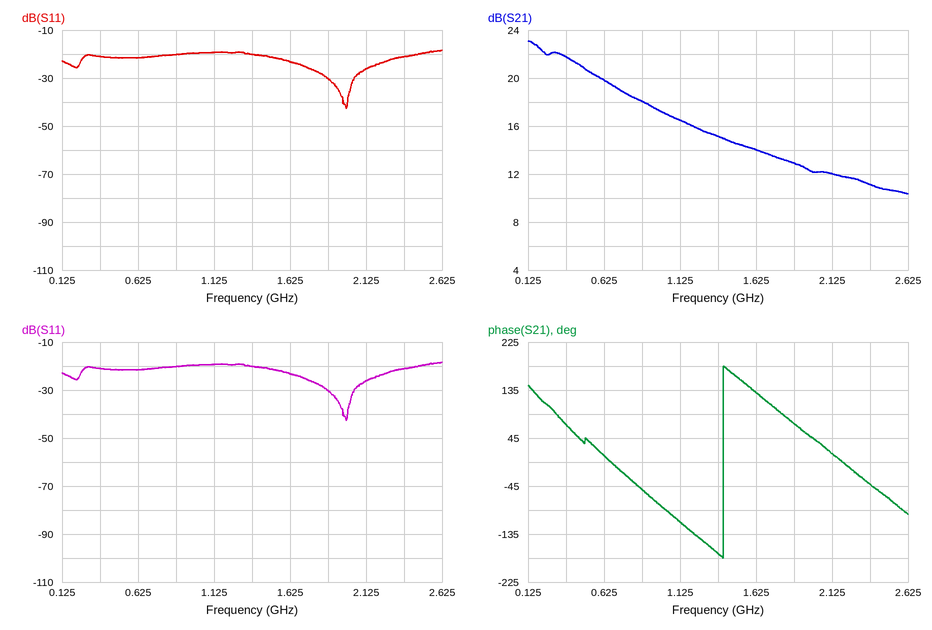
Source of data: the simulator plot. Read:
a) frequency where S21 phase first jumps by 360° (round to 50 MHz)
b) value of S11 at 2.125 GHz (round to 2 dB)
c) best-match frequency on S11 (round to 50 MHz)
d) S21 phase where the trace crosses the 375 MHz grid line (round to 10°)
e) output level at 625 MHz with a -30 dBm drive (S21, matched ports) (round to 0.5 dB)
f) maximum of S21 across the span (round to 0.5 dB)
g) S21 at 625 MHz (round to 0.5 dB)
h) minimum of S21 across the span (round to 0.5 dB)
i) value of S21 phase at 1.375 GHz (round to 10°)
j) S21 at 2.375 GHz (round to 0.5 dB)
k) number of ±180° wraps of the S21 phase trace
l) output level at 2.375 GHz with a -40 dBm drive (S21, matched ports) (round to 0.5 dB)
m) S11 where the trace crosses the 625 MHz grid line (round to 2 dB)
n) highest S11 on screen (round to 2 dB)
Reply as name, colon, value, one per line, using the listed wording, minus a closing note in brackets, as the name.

frequency where S21 phase first jumps by 360°: 1.40 GHz
value of S11 at 2.125 GHz: -26 dB
best-match frequency on S11: 2.00 GHz
S21 phase where the trace crosses the 375 MHz grid line: 70°
output level at 625 MHz with a -30 dBm drive (S21, matched ports): -10.0 dBm
maximum of S21 across the span: 23.0 dB
S21 at 625 MHz: 20.0 dB
minimum of S21 across the span: 10.5 dB
value of S21 phase at 1.375 GHz: -170°
S21 at 2.375 GHz: 11.0 dB
number of ±180° wraps of the S21 phase trace: 1
output level at 2.375 GHz with a -40 dBm drive (S21, matched ports): -29.0 dBm
S11 where the trace crosses the 625 MHz grid line: -22 dB
highest S11 on screen: -18 dB
